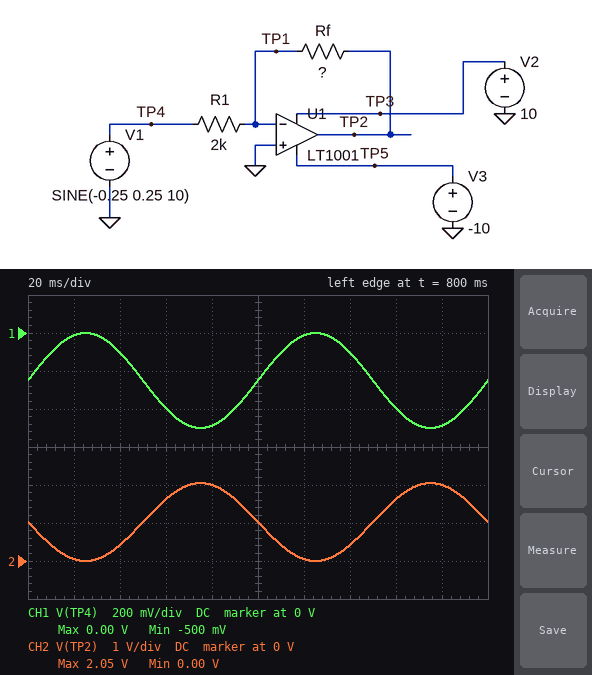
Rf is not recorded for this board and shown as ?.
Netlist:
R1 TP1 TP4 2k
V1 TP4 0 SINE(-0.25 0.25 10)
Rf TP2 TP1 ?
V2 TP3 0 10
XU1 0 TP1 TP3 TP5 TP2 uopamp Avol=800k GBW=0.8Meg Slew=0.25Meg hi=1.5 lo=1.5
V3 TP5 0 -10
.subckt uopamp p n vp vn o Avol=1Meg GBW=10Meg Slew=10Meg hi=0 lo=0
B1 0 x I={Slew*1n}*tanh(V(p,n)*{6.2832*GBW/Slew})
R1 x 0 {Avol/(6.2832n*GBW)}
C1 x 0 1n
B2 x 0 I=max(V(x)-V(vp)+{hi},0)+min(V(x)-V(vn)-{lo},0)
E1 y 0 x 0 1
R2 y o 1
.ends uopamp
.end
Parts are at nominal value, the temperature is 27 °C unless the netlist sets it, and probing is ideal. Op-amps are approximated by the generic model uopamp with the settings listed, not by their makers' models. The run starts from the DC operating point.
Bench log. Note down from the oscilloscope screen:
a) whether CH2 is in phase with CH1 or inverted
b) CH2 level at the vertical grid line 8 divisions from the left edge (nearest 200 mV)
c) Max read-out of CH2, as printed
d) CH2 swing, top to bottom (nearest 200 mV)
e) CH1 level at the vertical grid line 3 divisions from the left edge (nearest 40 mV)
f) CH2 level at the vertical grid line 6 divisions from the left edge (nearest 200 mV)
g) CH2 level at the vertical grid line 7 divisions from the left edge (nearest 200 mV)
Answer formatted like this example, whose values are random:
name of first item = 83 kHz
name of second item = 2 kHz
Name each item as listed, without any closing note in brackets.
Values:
whether CH2 is in phase with CH1 or inverted = inverted
CH2 level at the vertical grid line 8 divisions from the left edge = 1.6 V
Max read-out of CH2, as printed = 2.05 V
CH2 swing, top to bottom = 2.0 V
CH1 level at the vertical grid line 3 divisions from the left edge = -400 mV
CH2 level at the vertical grid line 6 divisions from the left edge = 0 V
CH2 level at the vertical grid line 7 divisions from the left edge = 400 mV
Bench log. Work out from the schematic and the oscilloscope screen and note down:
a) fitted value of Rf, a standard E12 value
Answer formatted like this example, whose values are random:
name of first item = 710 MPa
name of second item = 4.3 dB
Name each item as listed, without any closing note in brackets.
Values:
fitted value of Rf, a standard E12 value = 8.2 kΩ
